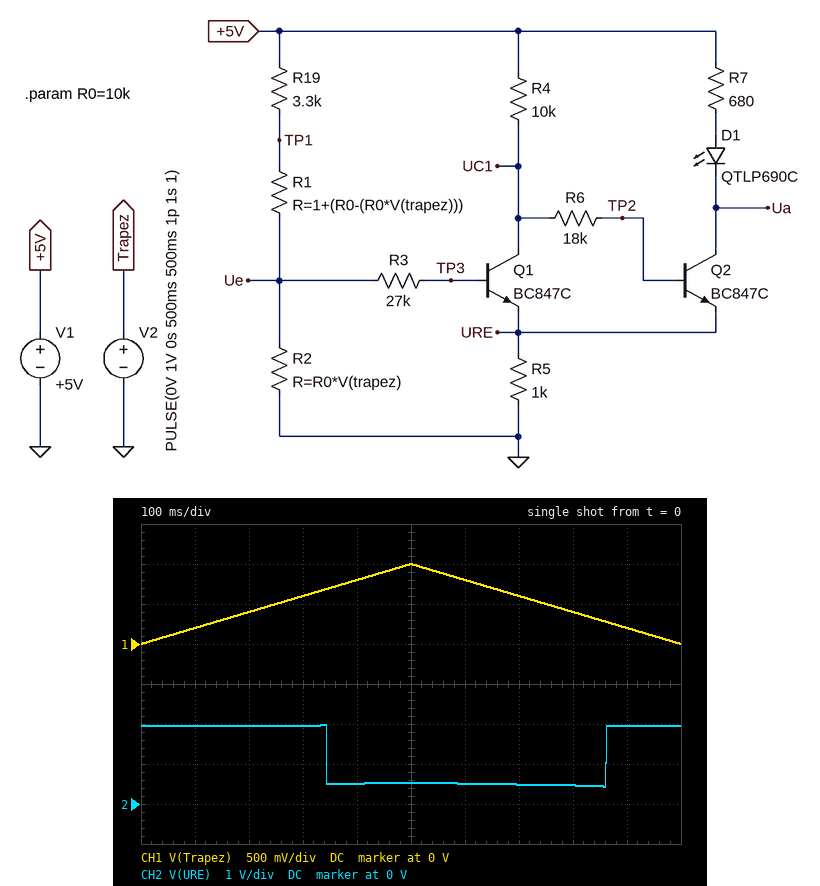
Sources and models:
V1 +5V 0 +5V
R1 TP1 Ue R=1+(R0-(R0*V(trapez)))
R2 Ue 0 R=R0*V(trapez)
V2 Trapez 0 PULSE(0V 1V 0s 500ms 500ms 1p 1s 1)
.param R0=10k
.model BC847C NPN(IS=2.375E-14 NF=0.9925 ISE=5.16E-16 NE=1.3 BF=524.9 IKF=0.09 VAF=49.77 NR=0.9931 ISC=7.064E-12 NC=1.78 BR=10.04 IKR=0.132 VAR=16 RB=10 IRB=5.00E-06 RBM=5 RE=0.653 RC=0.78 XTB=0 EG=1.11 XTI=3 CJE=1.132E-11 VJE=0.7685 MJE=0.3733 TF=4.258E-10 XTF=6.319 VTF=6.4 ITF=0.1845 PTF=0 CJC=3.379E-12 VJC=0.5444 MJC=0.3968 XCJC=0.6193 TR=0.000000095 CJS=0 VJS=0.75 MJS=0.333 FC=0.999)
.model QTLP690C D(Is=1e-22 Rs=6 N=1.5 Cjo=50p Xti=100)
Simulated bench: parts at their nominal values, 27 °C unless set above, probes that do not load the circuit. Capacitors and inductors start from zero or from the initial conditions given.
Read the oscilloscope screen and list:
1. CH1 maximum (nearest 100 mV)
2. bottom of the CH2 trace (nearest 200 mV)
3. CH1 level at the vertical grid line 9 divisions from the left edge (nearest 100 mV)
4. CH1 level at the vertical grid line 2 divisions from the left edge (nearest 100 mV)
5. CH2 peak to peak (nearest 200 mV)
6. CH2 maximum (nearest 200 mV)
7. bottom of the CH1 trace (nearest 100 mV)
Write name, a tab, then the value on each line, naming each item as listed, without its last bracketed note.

CH1 maximum	1.0 V
bottom of the CH2 trace	400 mV
CH1 level at the vertical grid line 9 divisions from the left edge	200 mV
CH1 level at the vertical grid line 2 divisions from the left edge	400 mV
CH2 peak to peak	1.6 V
CH2 maximum	2.0 V
bottom of the CH1 trace	0 V
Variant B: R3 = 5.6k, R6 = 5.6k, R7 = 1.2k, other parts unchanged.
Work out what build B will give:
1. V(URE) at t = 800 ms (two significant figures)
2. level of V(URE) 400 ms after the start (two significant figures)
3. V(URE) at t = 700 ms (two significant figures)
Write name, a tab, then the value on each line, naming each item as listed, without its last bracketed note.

V(URE) at t = 800 ms	490 mV
level of V(URE) 400 ms after the start	630 mV
V(URE) at t = 700 ms	560 mV
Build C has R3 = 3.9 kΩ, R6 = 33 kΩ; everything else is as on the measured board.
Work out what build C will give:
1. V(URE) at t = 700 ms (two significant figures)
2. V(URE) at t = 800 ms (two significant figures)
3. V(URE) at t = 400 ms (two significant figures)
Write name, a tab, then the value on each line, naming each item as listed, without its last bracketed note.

V(URE) at t = 700 ms	580 mV
V(URE) at t = 800 ms	500 mV
V(URE) at t = 400 ms	670 mV
